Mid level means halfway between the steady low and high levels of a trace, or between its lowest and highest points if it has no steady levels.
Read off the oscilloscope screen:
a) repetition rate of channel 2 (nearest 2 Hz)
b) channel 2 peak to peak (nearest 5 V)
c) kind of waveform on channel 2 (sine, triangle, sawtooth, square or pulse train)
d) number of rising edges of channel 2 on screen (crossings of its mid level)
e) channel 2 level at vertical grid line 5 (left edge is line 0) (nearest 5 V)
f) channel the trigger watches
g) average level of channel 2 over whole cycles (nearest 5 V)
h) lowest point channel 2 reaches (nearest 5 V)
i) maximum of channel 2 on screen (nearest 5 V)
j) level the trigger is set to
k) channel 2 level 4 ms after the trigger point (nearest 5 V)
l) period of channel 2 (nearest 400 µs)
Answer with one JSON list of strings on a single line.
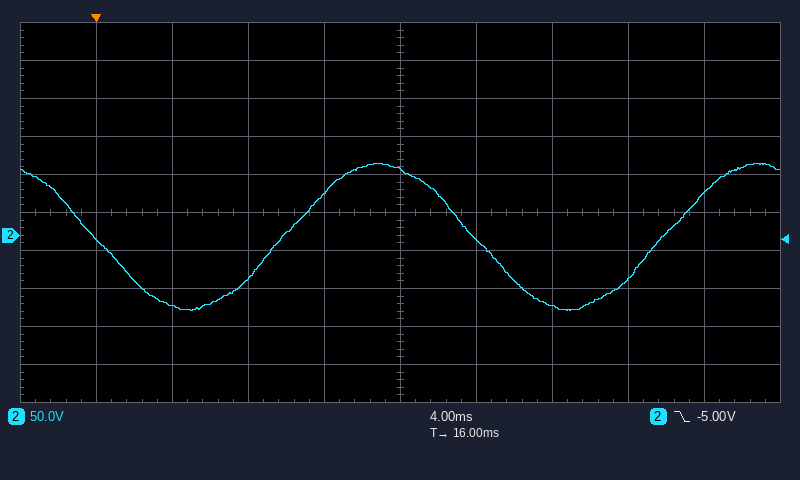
["50 Hz", "195 V", "sine", "2", "85 V", "channel 2", "0 V", "-100 V", "95 V", "-5.00 V", "-95 V", "20.0 ms"]
